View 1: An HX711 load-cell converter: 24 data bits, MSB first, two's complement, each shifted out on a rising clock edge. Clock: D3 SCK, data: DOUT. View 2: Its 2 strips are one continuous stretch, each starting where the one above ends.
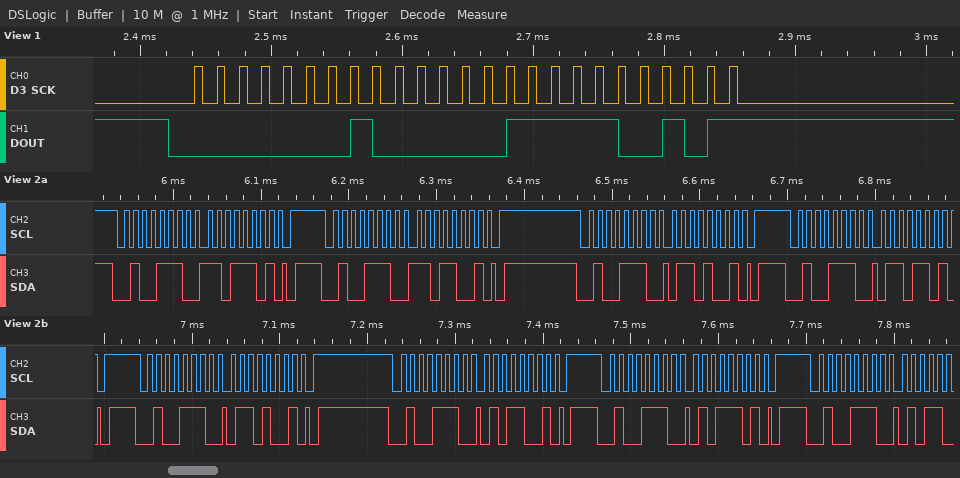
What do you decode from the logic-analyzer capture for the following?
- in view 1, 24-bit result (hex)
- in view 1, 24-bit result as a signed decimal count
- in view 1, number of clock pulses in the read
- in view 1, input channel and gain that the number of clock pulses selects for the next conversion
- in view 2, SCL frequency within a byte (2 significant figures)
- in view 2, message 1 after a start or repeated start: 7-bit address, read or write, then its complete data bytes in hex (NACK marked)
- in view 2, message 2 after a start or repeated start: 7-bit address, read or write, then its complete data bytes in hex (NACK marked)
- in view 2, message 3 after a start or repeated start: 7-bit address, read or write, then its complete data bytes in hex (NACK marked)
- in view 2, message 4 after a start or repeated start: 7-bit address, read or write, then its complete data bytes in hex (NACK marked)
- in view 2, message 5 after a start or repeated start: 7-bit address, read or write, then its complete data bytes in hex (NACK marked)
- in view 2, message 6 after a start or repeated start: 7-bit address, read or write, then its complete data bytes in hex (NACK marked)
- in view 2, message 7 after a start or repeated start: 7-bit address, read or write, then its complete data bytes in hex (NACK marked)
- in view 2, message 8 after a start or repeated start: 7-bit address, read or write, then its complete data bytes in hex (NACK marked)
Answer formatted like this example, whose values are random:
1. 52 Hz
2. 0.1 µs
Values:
1. 0x0103E5
2. 66533
3. 25
4. channel A, gain 128
5. 100 kHz
6. 0x27 write: DD
7. 0x27 write: D9
8. 0x27 write: 69
9. 0x27 write: 6D
10. 0x27 write: 69
11. 0x27 write: 59
12. 0x27 write: 5D
13. 0x27 write
